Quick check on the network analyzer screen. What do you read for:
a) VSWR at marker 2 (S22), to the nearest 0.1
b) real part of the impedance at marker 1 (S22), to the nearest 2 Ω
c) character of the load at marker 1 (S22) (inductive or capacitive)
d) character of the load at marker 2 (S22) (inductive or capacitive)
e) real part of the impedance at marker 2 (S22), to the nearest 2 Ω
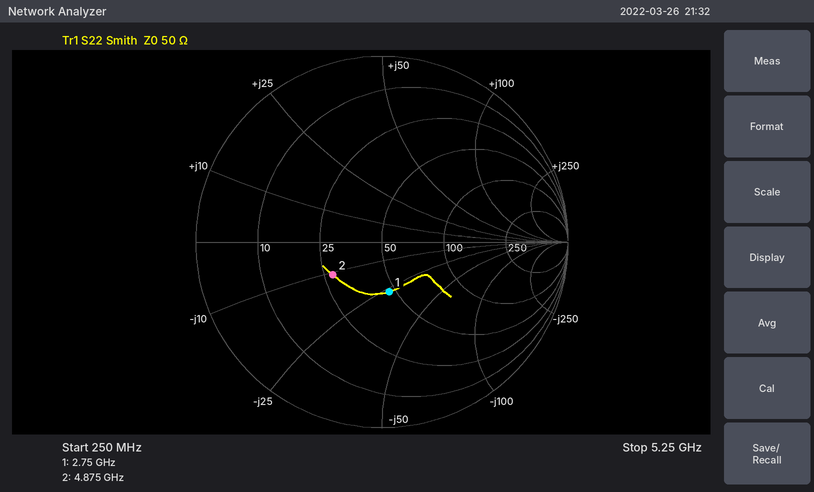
1.9
46 Ω
capacitive
capacitive
28 Ω
